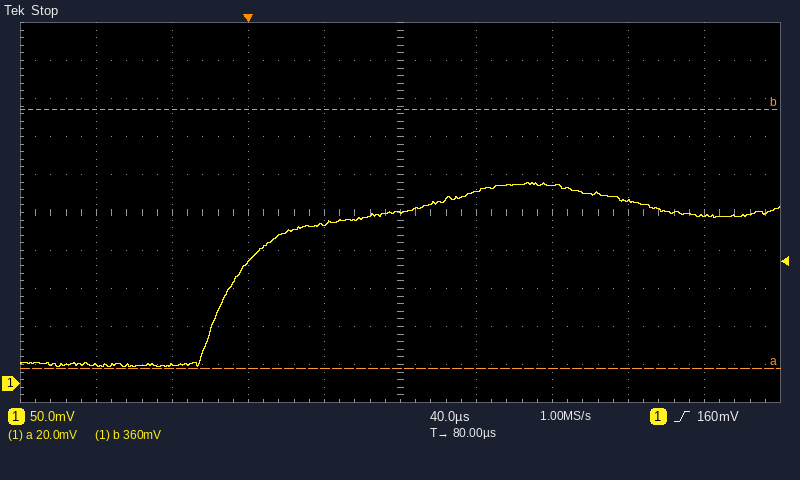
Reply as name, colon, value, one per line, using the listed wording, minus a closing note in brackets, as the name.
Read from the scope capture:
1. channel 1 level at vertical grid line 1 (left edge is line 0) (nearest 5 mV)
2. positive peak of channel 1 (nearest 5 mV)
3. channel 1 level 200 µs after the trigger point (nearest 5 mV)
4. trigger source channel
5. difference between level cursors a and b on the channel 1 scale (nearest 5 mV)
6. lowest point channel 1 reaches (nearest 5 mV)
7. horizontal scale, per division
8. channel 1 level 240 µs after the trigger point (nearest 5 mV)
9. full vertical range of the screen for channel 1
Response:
channel 1 level at vertical grid line 1 (left edge is line 0): 25 mV
positive peak of channel 1: 265 mV
channel 1 level 200 µs after the trigger point: 240 mV
trigger source channel: channel 1
difference between level cursors a and b on the channel 1 scale: 340 mV
lowest point channel 1 reaches: 20 mV
horizontal scale, per division: 40 µs
channel 1 level 240 µs after the trigger point: 220 mV
full vertical range of the screen for channel 1: 500 mV
